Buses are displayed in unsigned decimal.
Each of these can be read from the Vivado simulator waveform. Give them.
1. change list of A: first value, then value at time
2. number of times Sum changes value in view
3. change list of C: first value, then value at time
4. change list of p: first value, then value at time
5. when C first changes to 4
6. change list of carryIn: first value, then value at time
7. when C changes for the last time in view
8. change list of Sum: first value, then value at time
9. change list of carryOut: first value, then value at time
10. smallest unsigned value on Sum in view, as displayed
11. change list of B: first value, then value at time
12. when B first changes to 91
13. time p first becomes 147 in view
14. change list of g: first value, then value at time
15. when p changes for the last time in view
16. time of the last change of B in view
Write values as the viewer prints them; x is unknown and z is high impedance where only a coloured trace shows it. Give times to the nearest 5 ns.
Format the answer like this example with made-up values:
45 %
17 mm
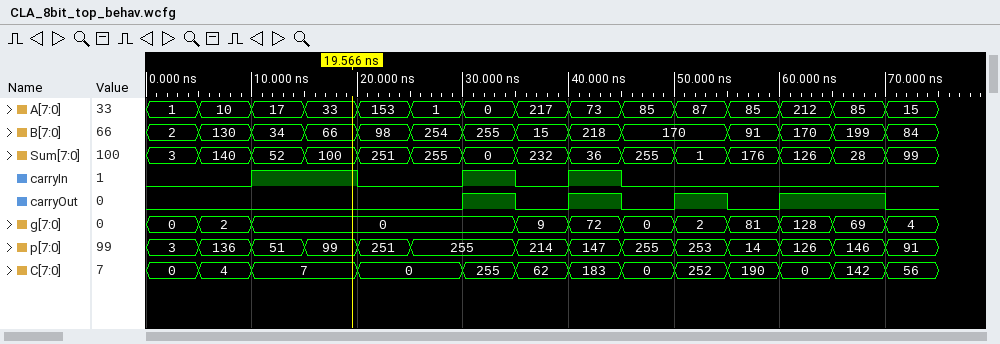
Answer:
1, 10 at 5 ns, 17 at 10 ns, 33 at 15 ns, 153 at 20 ns, 1 at 25 ns, 0 at 30 ns, 217 at 35 ns, 73 at 40 ns, 85 at 45 ns, 87 at 50 ns, 85 at 55 ns, 212 at 60 ns, 85 at 65 ns, 15 at 70 ns
14
0, 4 at 5 ns, 7 at 10 ns, 0 at 20 ns, 255 at 30 ns, 62 at 35 ns, 183 at 40 ns, 0 at 45 ns, 252 at 50 ns, 190 at 55 ns, 0 at 60 ns, 142 at 65 ns, 56 at 70 ns
3, 136 at 5 ns, 51 at 10 ns, 99 at 15 ns, 251 at 20 ns, 255 at 25 ns, 214 at 35 ns, 147 at 40 ns, 255 at 45 ns, 253 at 50 ns, 14 at 55 ns, 126 at 60 ns, 146 at 65 ns, 91 at 70 ns
5 ns
0, 1 at 10 ns, 0 at 20 ns, 1 at 30 ns, 0 at 35 ns, 1 at 40 ns, 0 at 45 ns
70 ns
3, 140 at 5 ns, 52 at 10 ns, 100 at 15 ns, 251 at 20 ns, 255 at 25 ns, 0 at 30 ns, 232 at 35 ns, 36 at 40 ns, 255 at 45 ns, 1 at 50 ns, 176 at 55 ns, 126 at 60 ns, 28 at 65 ns, 99 at 70 ns
0, 1 at 30 ns, 0 at 35 ns, 1 at 40 ns, 0 at 45 ns, 1 at 50 ns, 0 at 55 ns, 1 at 60 ns, 0 at 70 ns
0
2, 130 at 5 ns, 34 at 10 ns, 66 at 15 ns, 98 at 20 ns, 254 at 25 ns, 255 at 30 ns, 15 at 35 ns, 218 at 40 ns, 170 at 45 ns, 91 at 55 ns, 170 at 60 ns, 199 at 65 ns, 84 at 70 ns
55 ns
40 ns
0, 2 at 5 ns, 0 at 10 ns, 9 at 35 ns, 72 at 40 ns, 0 at 45 ns, 2 at 50 ns, 81 at 55 ns, 128 at 60 ns, 69 at 65 ns, 4 at 70 ns
70 ns
70 ns
